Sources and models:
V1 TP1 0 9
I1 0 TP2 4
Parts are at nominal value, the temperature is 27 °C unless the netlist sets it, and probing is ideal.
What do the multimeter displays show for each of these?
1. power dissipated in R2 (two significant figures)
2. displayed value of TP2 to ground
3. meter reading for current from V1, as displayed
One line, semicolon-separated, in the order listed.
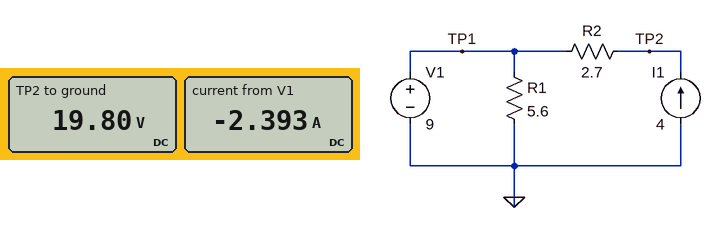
43 W; 19.80 V; -2.393 A
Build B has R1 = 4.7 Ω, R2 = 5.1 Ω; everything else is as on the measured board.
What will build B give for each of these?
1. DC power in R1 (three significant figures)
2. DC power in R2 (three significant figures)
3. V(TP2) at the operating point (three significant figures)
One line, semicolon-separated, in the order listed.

17.2 W; 81.6 W; 29.4 V
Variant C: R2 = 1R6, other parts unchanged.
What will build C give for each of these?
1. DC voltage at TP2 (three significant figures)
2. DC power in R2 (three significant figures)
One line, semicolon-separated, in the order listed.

15.4 V; 25.6 W
